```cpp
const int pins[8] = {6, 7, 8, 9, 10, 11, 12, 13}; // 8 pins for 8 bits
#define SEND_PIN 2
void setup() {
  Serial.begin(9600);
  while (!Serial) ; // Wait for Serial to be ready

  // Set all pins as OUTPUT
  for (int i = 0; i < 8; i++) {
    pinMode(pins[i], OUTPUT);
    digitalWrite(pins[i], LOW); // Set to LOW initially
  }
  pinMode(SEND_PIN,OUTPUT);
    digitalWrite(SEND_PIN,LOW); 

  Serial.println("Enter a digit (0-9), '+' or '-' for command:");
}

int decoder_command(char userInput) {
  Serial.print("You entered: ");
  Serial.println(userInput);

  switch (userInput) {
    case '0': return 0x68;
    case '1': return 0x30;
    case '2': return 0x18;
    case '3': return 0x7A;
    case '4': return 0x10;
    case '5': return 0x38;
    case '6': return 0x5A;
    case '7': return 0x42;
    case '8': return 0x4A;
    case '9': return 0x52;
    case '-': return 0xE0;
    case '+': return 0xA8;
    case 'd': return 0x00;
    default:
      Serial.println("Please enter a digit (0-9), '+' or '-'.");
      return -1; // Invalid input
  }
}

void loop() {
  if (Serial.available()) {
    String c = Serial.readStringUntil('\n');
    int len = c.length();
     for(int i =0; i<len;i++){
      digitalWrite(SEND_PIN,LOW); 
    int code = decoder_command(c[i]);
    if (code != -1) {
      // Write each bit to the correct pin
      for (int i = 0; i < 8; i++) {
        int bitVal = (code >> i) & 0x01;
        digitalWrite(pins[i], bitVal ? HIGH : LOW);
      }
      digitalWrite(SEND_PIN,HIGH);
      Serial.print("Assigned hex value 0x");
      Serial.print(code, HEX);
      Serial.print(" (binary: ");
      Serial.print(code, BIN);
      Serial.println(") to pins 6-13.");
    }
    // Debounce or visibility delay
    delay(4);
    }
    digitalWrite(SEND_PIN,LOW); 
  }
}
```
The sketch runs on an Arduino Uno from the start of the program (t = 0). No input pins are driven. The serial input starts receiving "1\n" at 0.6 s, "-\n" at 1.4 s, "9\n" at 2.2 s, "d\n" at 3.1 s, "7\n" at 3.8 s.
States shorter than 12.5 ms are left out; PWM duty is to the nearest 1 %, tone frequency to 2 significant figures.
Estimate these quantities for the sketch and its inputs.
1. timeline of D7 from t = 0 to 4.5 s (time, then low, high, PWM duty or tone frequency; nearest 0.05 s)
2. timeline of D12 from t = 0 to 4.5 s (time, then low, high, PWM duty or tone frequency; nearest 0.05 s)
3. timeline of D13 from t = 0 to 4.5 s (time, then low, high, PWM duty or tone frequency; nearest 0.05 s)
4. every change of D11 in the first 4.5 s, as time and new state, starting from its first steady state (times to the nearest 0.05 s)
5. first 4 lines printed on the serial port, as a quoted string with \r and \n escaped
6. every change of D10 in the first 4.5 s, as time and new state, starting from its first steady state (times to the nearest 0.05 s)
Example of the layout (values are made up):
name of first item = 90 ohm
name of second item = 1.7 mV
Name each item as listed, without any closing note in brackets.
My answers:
timeline of D7 from t = 0 to 4.5 s = 0 s low; 2.2 s high; 3.1 s low; 3.8 s high
timeline of D12 from t = 0 to 4.5 s = 0 s low; 1.4 s high; 3.1 s low; 3.8 s high
timeline of D13 from t = 0 to 4.5 s = 0 s low; 1.4 s high; 2.2 s low
every change of D11 in the first 4.5 s, as time and new state, starting from its first steady state = 0 s low; 0.6 s high; 2.2 s low
first 4 lines printed on the serial port, as a quoted string with \r and \n escaped = "Enter a digit (0-9), '+' or '-' for command:\r\nYou entered: 1\r\nAssigned hex value 0x30 (binary: 110000) to pins 6-13.\r\nYou entered: -\r\n"
every change of D10 in the first 4.5 s, as time and new state, starting from its first steady state = 0 s low; 0.6 s high; 1.4 s low; 2.2 s high; 3.1 s low
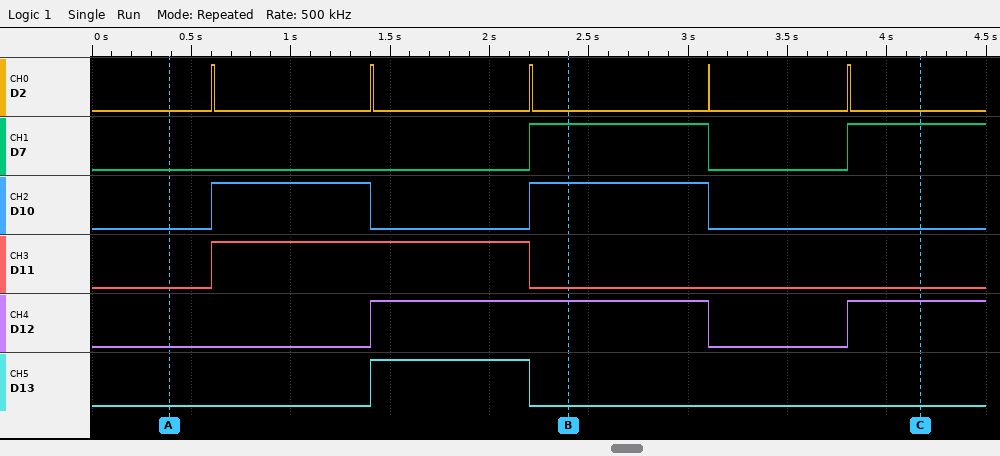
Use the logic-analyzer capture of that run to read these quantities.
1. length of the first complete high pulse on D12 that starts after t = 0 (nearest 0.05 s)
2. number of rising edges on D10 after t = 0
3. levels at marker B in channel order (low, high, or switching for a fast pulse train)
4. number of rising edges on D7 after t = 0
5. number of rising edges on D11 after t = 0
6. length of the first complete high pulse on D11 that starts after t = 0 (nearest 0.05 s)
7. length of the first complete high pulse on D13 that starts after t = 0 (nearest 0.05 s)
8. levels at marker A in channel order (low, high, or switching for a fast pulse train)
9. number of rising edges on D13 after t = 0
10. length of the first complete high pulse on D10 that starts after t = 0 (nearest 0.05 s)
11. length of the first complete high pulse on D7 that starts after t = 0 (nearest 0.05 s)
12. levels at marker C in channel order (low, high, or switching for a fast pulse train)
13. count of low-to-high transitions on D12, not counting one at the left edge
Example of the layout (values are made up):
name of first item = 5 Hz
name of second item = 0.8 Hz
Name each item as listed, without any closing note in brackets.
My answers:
length of the first complete high pulse on D12 that starts after t = 0 = 1.70 s
number of rising edges on D10 after t = 0 = 2
levels at marker B in channel order = D2 low, D7 high, D10 high, D11 low, D12 high, D13 low
number of rising edges on D7 after t = 0 = 2
number of rising edges on D11 after t = 0 = 1
length of the first complete high pulse on D11 that starts after t = 0 = 1.60 s
length of the first complete high pulse on D13 that starts after t = 0 = 0.80 s
levels at marker A in channel order = D2 low, D7 low, D10 low, D11 low, D12 low, D13 low
number of rising edges on D13 after t = 0 = 1
length of the first complete high pulse on D10 that starts after t = 0 = 0.80 s
length of the first complete high pulse on D7 that starts after t = 0 = 0.90 s
levels at marker C in channel order = D2 low, D7 high, D10 low, D11 low, D12 high, D13 low
count of low-to-high transitions on D12, not counting one at the left edge = 2
